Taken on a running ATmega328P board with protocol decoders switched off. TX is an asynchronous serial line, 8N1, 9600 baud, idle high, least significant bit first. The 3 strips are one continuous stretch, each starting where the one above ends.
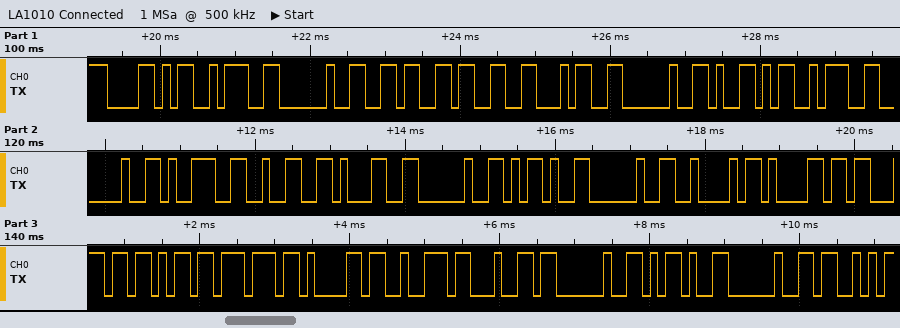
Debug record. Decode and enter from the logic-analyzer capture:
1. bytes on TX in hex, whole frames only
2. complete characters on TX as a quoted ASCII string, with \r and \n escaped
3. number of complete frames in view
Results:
58 3A 20 36 33 34 20 59 3A 20 39 32 31 20 2D 20 42 61 63 6B 77 61 72 64 20 2D 20 53
"X: 634 Y: 921 - Backward - S"
28
